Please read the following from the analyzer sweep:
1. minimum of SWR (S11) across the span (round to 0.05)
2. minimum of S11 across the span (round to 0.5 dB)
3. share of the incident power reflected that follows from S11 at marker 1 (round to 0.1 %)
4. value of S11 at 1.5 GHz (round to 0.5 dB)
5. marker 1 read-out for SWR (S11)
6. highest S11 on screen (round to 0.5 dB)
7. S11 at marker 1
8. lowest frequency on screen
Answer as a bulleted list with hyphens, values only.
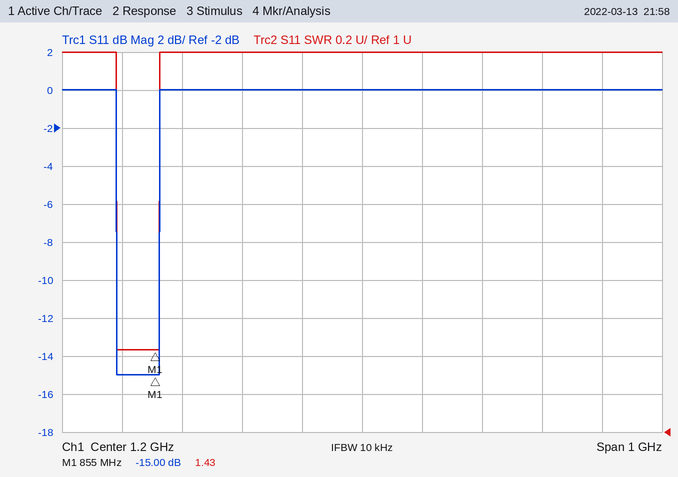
- 1.45
- -15.0 dB
- 3.2 %
- 0.0 dB
- 1.43
- 0.0 dB
- -15.00 dB
- 700 MHz
